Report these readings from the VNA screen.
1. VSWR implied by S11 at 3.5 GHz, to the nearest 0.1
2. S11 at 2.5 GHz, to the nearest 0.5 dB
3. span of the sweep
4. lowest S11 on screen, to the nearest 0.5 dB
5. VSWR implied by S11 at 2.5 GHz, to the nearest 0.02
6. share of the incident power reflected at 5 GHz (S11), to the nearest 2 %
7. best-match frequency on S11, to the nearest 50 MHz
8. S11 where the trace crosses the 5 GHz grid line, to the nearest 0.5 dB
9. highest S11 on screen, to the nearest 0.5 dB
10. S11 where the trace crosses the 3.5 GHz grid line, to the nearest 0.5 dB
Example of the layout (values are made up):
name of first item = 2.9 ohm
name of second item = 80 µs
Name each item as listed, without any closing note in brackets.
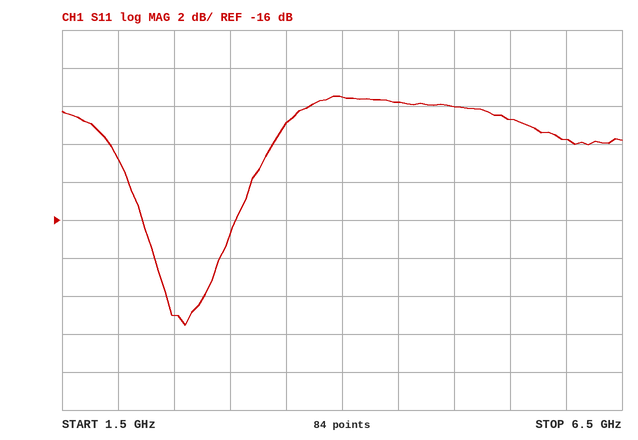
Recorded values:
VSWR implied by S11 at 3.5 GHz, to the nearest 0.1 = 1.8
S11 at 2.5 GHz, to the nearest 0.5 dB = -21.0 dB
span of the sweep = 5 GHz
lowest S11 on screen, to the nearest 0.5 dB = -21.5 dB
VSWR implied by S11 at 2.5 GHz, to the nearest 0.02 = 1.20
share of the incident power reflected at 5 GHz (S11), to the nearest 2 % = 10 %
best-match frequency on S11, to the nearest 50 MHz = 2.60 GHz
S11 where the trace crosses the 5 GHz grid line, to the nearest 0.5 dB = -10.0 dB
highest S11 on screen, to the nearest 0.5 dB = -9.5 dB
S11 where the trace crosses the 3.5 GHz grid line, to the nearest 0.5 dB = -11.0 dB
